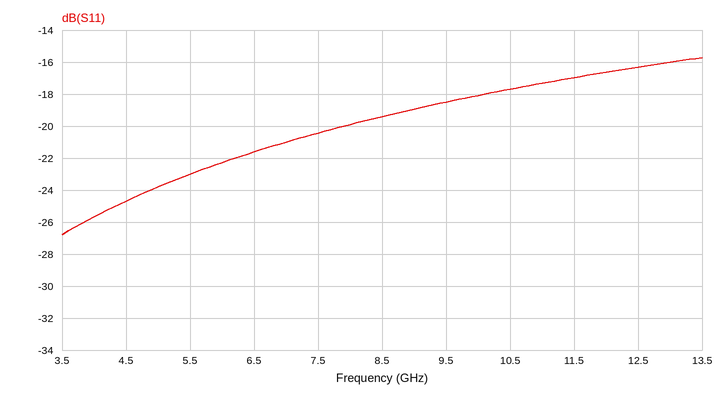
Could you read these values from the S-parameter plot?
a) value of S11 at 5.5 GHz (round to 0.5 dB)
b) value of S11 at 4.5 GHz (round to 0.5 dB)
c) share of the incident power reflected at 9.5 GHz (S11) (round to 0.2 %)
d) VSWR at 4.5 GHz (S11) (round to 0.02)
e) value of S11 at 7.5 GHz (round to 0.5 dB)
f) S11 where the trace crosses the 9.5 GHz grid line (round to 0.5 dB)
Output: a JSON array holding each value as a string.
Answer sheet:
["-23.0 dB", "-24.5 dB", "1.4 %", "1.12", "-20.5 dB", "-18.5 dB"]
